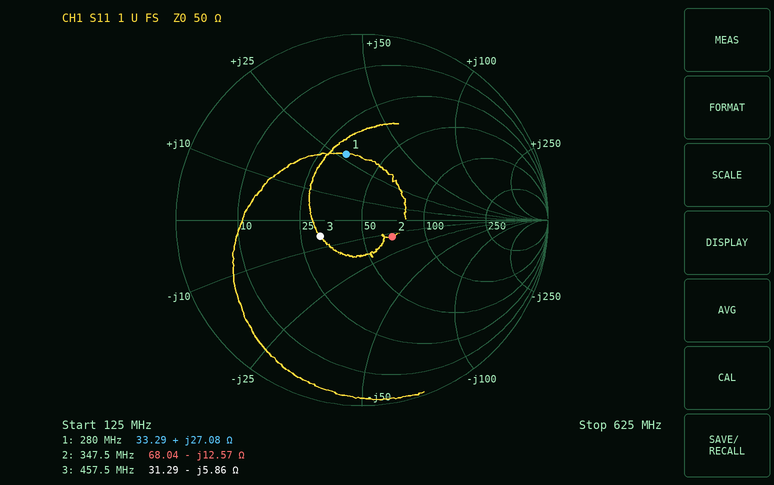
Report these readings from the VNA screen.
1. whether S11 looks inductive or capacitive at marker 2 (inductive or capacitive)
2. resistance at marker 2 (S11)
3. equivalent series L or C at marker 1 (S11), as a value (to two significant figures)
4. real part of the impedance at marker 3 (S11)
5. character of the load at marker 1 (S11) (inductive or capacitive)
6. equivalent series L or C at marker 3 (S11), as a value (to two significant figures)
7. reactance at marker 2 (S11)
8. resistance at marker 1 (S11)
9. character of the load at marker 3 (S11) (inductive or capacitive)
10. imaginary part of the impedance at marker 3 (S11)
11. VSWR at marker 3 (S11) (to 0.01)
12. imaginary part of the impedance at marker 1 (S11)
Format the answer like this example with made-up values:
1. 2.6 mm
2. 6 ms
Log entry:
1. capacitive
2. 68.04 Ω
3. 15 nH
4. 31.29 Ω
5. inductive
6. 59 pF
7. -12.57 Ω
8. 33.29 Ω
9. capacitive
10. -5.86 Ω
11. 1.63
12. +27.08 Ω
